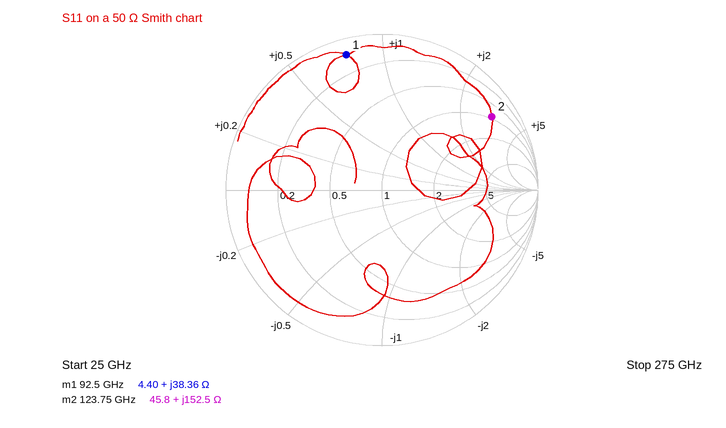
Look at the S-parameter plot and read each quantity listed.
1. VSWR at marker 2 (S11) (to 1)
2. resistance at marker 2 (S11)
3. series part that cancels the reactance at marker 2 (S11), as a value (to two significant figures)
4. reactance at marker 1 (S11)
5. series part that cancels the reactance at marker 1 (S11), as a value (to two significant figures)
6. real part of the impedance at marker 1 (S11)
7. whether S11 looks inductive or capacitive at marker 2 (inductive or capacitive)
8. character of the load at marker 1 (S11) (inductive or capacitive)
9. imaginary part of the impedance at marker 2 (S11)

12
45.8 Ω
8.4 fF
+38.36 Ω
45 fF
4.40 Ω
inductive
inductive
+152.5 Ω
